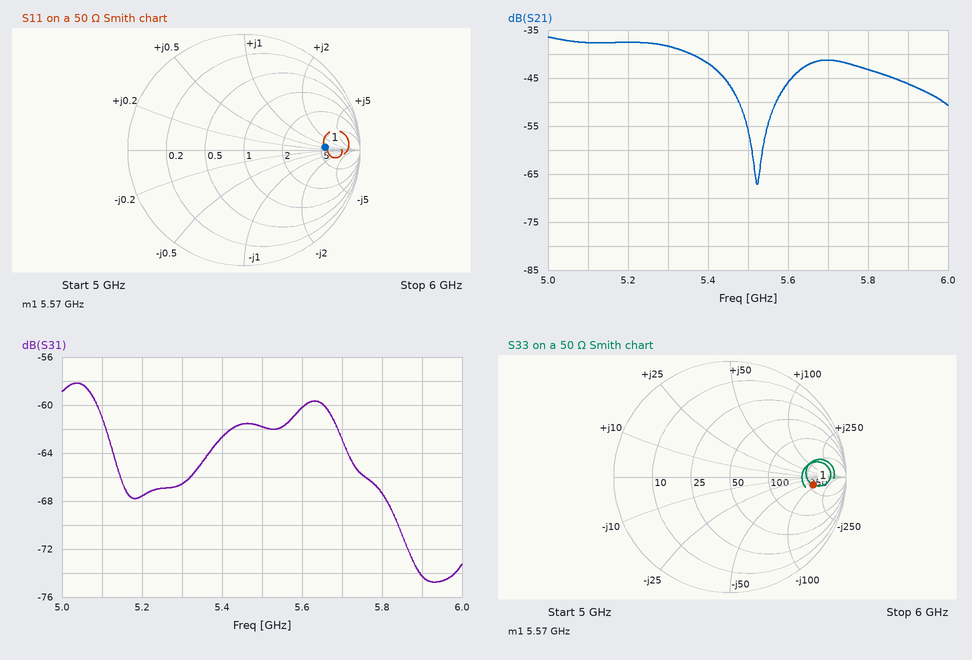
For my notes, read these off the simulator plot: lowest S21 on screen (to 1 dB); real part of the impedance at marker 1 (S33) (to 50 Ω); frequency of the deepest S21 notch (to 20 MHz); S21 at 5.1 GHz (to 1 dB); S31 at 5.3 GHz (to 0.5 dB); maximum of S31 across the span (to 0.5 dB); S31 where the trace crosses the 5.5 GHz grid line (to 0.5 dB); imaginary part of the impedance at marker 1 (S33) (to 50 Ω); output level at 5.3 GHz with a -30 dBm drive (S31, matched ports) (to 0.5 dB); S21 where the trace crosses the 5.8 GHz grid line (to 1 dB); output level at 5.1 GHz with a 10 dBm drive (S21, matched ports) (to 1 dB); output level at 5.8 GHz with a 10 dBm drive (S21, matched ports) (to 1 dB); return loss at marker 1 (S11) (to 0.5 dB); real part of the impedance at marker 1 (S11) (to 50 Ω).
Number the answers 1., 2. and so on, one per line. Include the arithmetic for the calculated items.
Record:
1. -67 dB
2. 300 Ω
3. 5.52 GHz
4. -38 dB
5. -66.5 dB
6. -58.0 dB
7. -62.0 dB
8. -100 Ω
9. -30 dBm + (-66.5 dB) = -96.5 dBm
10. -43 dB
11. 10 dBm + (-38 dB) = -28 dBm
12. 10 dBm + (-43 dB) = -33 dBm
13. 3.0 dB
14. 300 Ω
